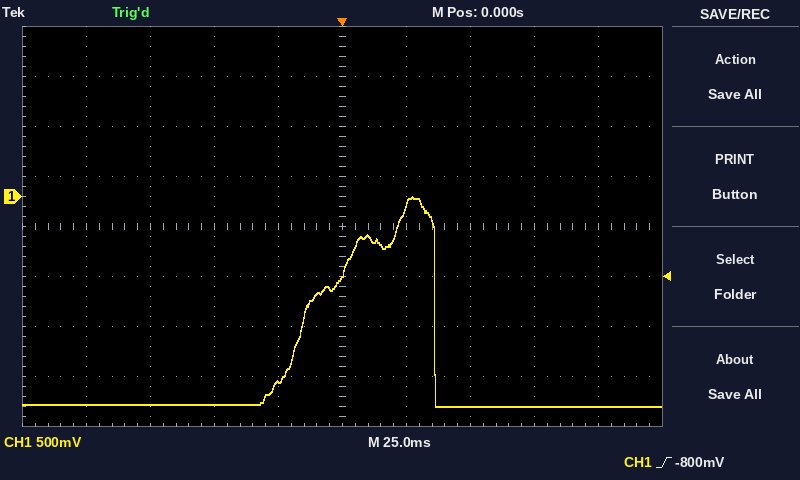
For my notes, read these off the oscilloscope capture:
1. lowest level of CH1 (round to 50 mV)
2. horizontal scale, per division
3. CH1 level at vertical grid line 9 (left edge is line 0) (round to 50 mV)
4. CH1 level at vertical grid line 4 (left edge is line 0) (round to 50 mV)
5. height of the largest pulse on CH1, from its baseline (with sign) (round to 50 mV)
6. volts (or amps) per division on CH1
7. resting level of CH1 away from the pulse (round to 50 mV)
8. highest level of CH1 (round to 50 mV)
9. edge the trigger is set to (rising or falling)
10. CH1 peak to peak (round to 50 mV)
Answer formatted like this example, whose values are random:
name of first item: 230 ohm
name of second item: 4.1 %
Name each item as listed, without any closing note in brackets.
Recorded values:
lowest level of CH1: -2.10 V
horizontal scale, per division: 25 ms
CH1 level at vertical grid line 9 (left edge is line 0): -2.10 V
CH1 level at vertical grid line 4 (left edge is line 0): -1.85 V
height of the largest pulse on CH1, from its baseline (with sign): +2.10 V
volts (or amps) per division on CH1: 500 mV
resting level of CH1 away from the pulse: -2.10 V
highest level of CH1: 0 mV
edge the trigger is set to: rising
CH1 peak to peak: 2.10 V
